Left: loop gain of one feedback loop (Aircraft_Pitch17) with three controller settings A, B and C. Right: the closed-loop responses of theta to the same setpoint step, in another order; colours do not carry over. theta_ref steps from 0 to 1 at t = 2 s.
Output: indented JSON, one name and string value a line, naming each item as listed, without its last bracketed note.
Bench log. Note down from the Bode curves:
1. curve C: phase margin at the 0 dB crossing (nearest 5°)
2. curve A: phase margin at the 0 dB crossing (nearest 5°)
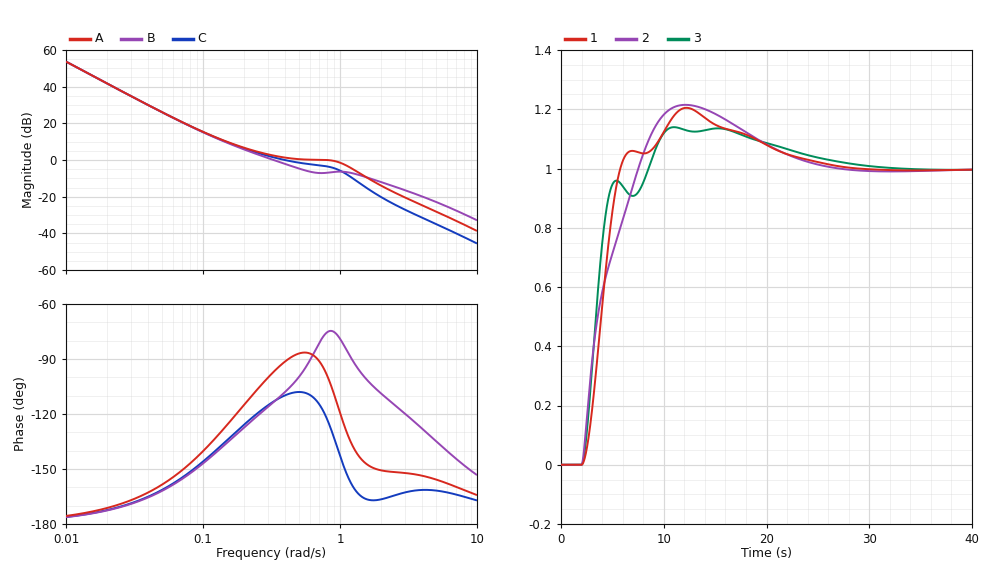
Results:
{
  "curve C: phase margin at the 0 dB crossing": "70°",
  "curve A: phase margin at the 0 dB crossing": "80°"
}
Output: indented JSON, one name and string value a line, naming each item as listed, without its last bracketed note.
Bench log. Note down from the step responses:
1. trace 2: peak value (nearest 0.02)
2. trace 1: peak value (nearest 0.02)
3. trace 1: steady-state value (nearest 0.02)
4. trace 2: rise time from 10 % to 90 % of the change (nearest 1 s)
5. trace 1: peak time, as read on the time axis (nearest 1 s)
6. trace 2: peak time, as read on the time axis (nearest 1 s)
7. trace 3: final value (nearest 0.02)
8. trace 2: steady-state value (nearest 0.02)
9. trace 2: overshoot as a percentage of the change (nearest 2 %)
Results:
{
  "trace 2: peak value": "1.22",
  "trace 1: peak value": "1.20",
  "trace 1: steady-state value": "1.00",
  "trace 2: rise time from 10 % to 90 % of the change": "4 s",
  "trace 1: peak time, as read on the time axis": "12 s",
  "trace 2: peak time, as read on the time axis": "12 s",
  "trace 3: final value": "1.00",
  "trace 2: steady-state value": "1.00",
  "trace 2: overshoot as a percentage of the change": "22 %"
}
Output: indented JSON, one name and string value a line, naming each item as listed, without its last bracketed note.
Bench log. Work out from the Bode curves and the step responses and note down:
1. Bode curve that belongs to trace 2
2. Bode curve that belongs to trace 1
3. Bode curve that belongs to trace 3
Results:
{
  "Bode curve that belongs to trace 2": "B",
  "Bode curve that belongs to trace 1": "C",
  "Bode curve that belongs to trace 3": "A"
}
